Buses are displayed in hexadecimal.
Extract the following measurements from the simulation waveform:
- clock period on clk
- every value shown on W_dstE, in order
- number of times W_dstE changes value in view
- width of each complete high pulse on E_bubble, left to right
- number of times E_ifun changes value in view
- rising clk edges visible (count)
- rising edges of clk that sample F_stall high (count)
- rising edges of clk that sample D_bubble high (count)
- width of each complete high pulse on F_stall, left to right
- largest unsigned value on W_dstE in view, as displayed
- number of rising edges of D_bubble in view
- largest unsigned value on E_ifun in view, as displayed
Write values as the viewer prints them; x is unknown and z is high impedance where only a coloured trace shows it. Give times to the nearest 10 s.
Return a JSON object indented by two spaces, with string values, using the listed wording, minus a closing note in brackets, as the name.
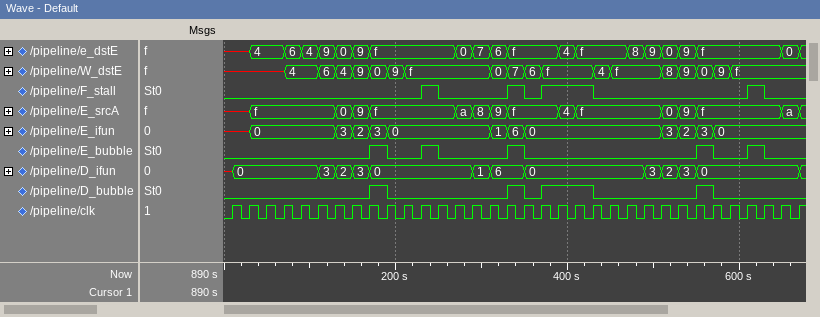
{
  "clock period on clk": "20 s",
  "every value shown on W_dstE, in order": "x, 4, 6, 4, 9, 0, 9, f, 0, 7, 6, f, 4, f, 8, 9, 0, 9, f",
  "number of times W_dstE changes value in view": "18",
  "width of each complete high pulse on E_bubble, left to right": "20 s, 20 s, 20 s, 20 s, 20 s",
  "number of times E_ifun changes value in view": "12",
  "rising clk edges visible": "34",
  "rising edges of clk that sample F_stall high": "6",
  "rising edges of clk that sample D_bubble high": "6",
  "width of each complete high pulse on F_stall, left to right": "20 s, 20 s, 60 s, 20 s",
  "largest unsigned value on W_dstE in view, as displayed": "f",
  "number of rising edges of D_bubble in view": "4",
  "largest unsigned value on E_ifun in view, as displayed": "6"
}
